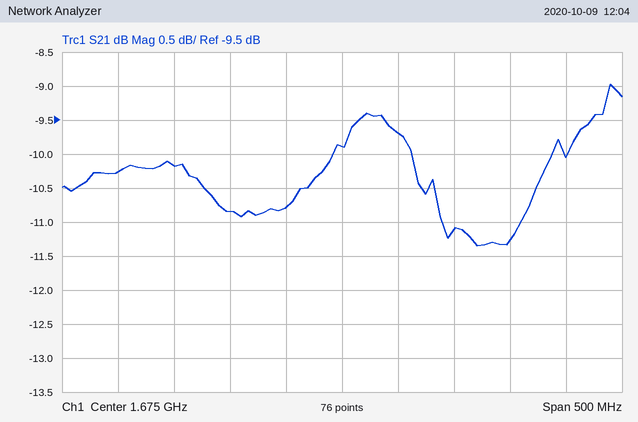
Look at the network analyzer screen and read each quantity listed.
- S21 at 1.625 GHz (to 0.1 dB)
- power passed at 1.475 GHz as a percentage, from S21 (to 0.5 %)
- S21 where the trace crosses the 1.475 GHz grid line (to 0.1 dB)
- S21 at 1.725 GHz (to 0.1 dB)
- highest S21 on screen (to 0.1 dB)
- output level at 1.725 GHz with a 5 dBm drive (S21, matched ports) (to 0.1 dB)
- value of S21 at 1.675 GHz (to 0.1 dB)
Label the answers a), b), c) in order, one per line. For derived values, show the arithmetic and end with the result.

a) -10.8 dB
b) 10^(-10.3/10) ≈ 9.33 %, so 9.5 % to the nearest 0.5 %
c) -10.3 dB
d) -9.7 dB
e) -9.0 dB
f) 5 dBm + (-9.7 dB) = -4.7 dBm
g) -9.9 dB
